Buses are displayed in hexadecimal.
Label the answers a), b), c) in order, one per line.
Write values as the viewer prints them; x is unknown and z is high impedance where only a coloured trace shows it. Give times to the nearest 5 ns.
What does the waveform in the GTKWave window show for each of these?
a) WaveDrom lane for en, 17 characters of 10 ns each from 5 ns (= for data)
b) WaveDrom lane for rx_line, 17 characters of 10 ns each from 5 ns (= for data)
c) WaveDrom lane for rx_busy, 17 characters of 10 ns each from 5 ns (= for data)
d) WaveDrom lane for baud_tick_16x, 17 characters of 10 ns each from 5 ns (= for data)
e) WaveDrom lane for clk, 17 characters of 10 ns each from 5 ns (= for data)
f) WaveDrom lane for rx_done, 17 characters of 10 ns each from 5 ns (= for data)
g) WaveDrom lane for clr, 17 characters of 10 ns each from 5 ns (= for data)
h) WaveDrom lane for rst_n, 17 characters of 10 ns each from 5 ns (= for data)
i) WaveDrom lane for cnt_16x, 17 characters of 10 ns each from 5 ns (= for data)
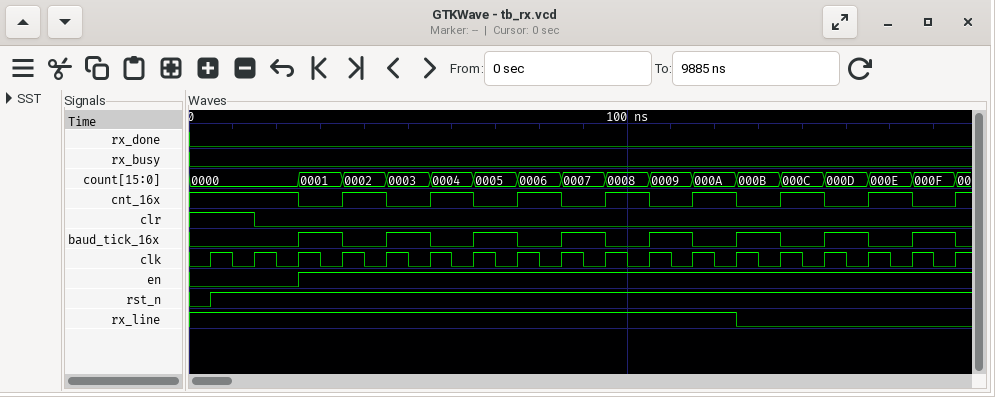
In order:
a) {name: 'en', wave: '0.1..............'}
b) {name: 'rx_line', wave: '1...........0....'}
c) {name: 'rx_busy', wave: '0................'}
d) {name: 'baud_tick_16x', wave: '0.101010101010101'}
e) {name: 'clk', wave: 'p................'}
f) {name: 'rx_done', wave: '0................'}
g) {name: 'clr', wave: '10...............'}
h) {name: 'rst_n', wave: '1................'}
i) {name: 'cnt_16x', wave: '1.010101010101010'}
